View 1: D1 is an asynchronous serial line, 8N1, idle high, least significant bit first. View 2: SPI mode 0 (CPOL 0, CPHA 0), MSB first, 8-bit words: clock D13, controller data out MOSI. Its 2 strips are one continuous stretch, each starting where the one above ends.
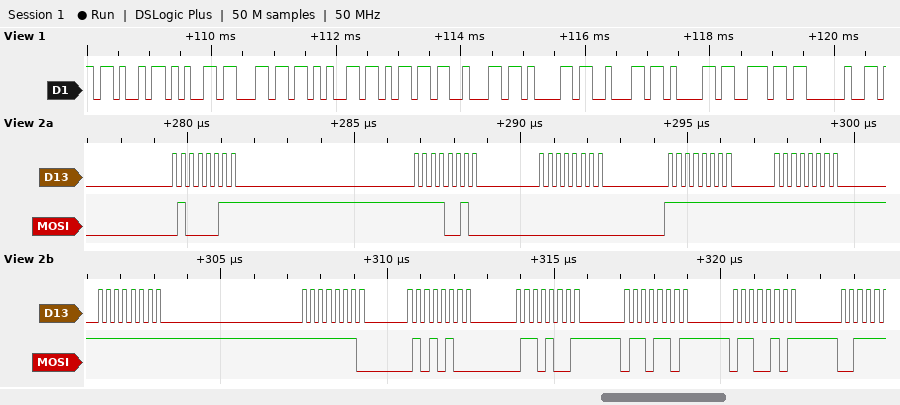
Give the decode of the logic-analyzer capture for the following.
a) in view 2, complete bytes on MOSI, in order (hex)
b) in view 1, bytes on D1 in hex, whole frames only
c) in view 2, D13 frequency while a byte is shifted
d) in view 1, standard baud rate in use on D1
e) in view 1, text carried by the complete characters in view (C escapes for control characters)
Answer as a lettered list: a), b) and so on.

a) 43 F2 00 FF FF FF FE 54 69 6D 65
b) 4B 65 6C 65 6D 62 61 62 61 6E 20
c) 4 MHz
d) 9600 baud
e) "Kelembaban "
